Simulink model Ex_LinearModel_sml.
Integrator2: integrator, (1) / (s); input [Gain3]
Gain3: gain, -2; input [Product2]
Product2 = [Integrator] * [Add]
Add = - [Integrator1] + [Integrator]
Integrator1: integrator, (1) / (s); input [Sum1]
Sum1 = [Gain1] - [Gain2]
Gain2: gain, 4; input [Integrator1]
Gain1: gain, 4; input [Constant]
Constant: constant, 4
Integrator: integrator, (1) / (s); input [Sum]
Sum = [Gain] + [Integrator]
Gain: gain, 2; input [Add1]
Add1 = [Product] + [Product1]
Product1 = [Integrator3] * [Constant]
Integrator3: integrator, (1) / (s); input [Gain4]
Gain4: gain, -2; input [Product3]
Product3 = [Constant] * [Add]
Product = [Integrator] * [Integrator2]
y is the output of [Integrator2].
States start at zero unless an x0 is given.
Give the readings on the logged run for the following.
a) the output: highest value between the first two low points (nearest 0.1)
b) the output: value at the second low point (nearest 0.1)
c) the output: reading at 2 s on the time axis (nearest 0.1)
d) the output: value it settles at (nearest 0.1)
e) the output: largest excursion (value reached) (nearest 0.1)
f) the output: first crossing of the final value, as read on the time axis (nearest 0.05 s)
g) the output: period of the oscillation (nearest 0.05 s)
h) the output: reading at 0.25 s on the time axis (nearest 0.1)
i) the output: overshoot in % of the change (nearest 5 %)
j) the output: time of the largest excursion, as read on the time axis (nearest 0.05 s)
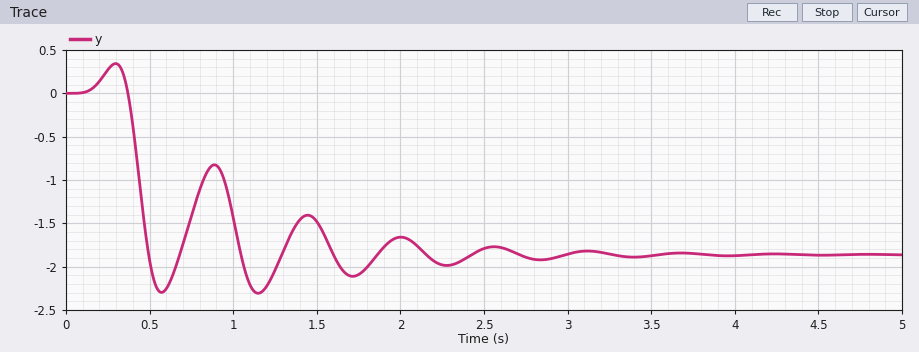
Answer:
-0.8
-2.3
-1.7
-1.9
-2.3
0.50 s
0.60 s
0.3
25 %
1.15 s
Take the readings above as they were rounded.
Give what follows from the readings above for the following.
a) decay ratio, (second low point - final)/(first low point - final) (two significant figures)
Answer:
1.0
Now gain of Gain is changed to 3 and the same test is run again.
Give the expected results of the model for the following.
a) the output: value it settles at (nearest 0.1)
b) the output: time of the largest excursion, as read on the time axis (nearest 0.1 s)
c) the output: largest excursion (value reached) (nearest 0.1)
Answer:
-1.3
1.0 s
-1.6
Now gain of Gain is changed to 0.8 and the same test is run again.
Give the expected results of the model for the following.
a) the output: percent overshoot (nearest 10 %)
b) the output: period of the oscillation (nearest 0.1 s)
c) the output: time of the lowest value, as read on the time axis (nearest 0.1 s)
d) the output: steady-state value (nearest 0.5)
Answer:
30 %
0.9 s
0.8 s
-4.0
